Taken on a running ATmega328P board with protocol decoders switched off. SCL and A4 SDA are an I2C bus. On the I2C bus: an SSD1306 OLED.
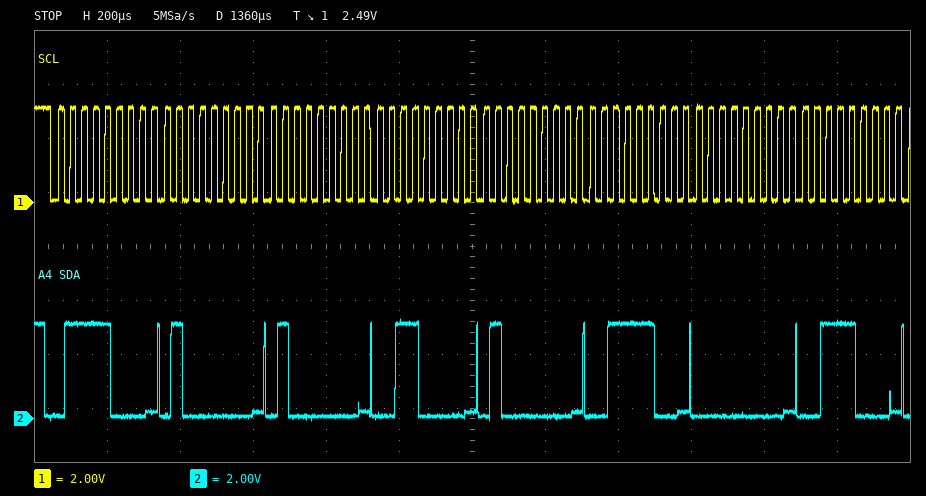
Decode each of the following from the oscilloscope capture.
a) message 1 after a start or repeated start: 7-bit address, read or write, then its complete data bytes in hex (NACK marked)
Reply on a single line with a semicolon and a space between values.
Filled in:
0x3C write: 40 40 30 40 3C 00 38
